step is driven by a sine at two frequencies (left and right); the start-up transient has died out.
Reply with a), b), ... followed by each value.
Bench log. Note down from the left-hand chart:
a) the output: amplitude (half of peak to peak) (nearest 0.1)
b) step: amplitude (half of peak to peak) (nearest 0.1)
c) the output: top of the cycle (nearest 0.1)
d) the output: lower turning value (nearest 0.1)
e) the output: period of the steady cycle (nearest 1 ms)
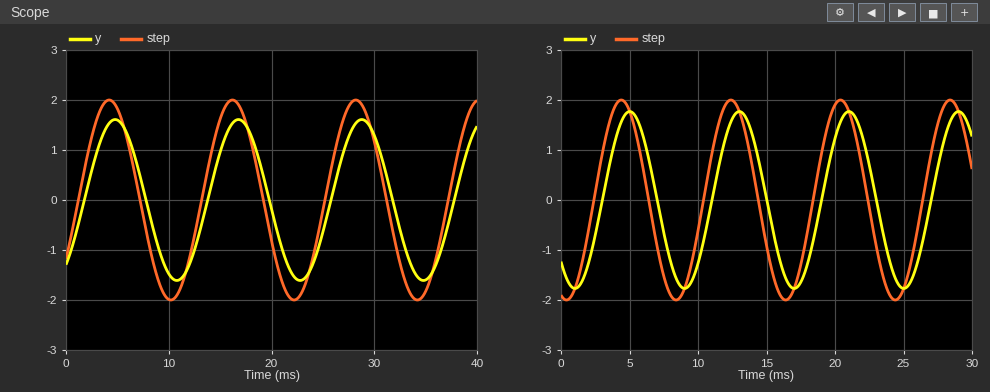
a) 1.6
b) 2.0
c) 1.6
d) -1.6
e) 12 ms
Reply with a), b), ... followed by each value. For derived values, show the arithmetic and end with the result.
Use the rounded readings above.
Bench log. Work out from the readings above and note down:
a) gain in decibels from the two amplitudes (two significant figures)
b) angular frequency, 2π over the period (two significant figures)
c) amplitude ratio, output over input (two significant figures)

a) 20 log10(1.6 / 2) = -1.9 dB
b) 2π / 12 = 0.52 rad/ms
c) 1.6 / 2 = 0.80
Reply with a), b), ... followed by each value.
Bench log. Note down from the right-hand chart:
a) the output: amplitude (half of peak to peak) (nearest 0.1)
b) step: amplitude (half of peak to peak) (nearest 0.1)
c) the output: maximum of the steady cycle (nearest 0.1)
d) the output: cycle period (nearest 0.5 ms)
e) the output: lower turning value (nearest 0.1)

a) 1.8
b) 2.0
c) 1.8
d) 8.0 ms
e) -1.8
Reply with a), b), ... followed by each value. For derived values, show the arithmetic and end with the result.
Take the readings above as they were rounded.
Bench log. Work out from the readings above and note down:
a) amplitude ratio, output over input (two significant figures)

a) 1.8 / 2 = 0.90
